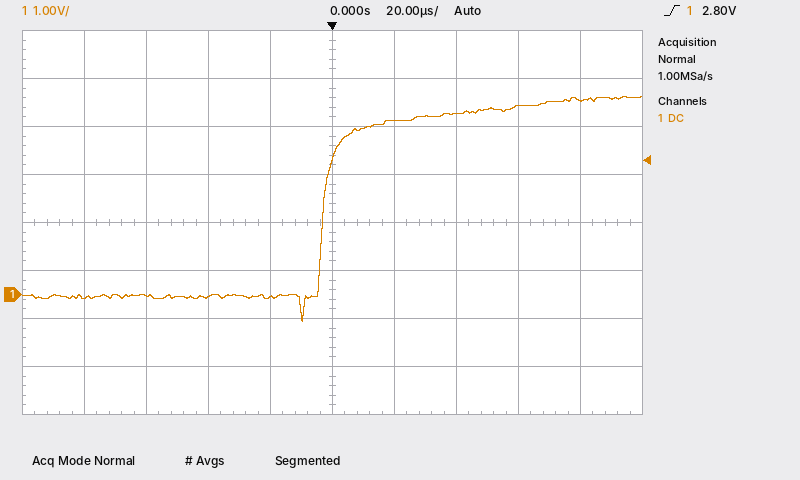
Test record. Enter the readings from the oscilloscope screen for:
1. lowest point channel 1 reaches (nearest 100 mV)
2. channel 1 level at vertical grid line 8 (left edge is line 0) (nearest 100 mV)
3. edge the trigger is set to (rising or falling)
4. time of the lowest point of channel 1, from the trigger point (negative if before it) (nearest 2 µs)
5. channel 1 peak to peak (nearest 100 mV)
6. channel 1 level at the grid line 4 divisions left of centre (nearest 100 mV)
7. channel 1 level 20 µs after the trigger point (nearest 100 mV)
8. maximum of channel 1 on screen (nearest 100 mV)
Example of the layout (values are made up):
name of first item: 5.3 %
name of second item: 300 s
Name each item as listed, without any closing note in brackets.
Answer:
lowest point channel 1 reaches: -600 mV
channel 1 level at vertical grid line 8 (left edge is line 0): 3.9 V
edge the trigger is set to: rising
time of the lowest point of channel 1, from the trigger point (negative if before it): -10 µs
channel 1 peak to peak: 4.7 V
channel 1 level at the grid line 4 divisions left of centre: -100 mV
channel 1 level 20 µs after the trigger point: 3.6 V
maximum of channel 1 on screen: 4.1 V
